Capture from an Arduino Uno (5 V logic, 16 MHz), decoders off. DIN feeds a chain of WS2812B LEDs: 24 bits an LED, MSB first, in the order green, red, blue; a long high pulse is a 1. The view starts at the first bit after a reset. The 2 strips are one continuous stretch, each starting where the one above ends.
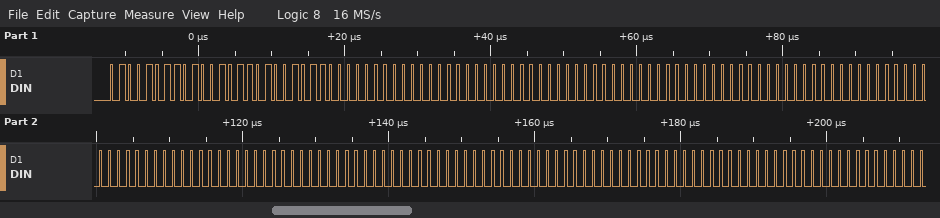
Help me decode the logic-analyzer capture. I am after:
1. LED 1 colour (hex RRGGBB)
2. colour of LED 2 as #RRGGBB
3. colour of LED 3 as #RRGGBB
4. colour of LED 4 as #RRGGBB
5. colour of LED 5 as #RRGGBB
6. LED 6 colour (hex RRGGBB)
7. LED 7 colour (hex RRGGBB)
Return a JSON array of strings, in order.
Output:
["#4B4B4B", "#000000", "#000000", "#000000", "#000000", "#000000", "#000000"]
